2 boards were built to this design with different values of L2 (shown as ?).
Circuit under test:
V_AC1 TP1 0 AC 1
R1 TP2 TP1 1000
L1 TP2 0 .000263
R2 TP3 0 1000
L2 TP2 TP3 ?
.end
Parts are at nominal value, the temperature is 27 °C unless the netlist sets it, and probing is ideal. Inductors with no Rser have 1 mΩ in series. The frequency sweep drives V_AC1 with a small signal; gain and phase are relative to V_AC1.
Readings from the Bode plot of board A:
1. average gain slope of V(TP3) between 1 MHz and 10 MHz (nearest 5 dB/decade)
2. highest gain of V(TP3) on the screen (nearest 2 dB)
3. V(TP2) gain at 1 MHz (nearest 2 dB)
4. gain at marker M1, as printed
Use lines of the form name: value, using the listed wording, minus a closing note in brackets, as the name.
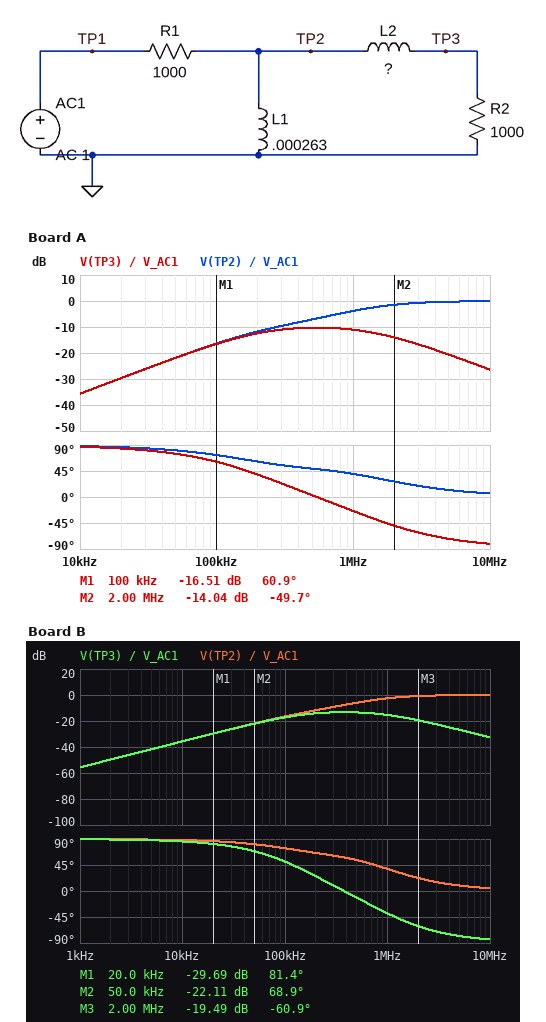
average gain slope of V(TP3) between 1 MHz and 10 MHz: -15 dB/decade
highest gain of V(TP3) on the screen: -10 dB
V(TP2) gain at 1 MHz: -4 dB
gain at marker M1, as printed: -16.51 dB
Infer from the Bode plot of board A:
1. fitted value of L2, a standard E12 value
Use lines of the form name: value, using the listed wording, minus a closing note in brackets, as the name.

fitted value of L2, a standard E12 value: 330 µH
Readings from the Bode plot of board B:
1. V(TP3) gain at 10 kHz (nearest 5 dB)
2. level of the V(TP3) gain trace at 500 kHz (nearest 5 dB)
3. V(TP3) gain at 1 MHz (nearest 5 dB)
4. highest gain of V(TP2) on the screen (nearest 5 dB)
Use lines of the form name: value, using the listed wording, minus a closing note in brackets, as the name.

V(TP3) gain at 10 kHz: -35 dB
level of the V(TP3) gain trace at 500 kHz: -15 dB
V(TP3) gain at 1 MHz: -15 dB
highest gain of V(TP2) on the screen: 0 dB
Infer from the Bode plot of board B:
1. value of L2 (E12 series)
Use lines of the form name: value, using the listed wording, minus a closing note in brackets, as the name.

value of L2: 680 µH
